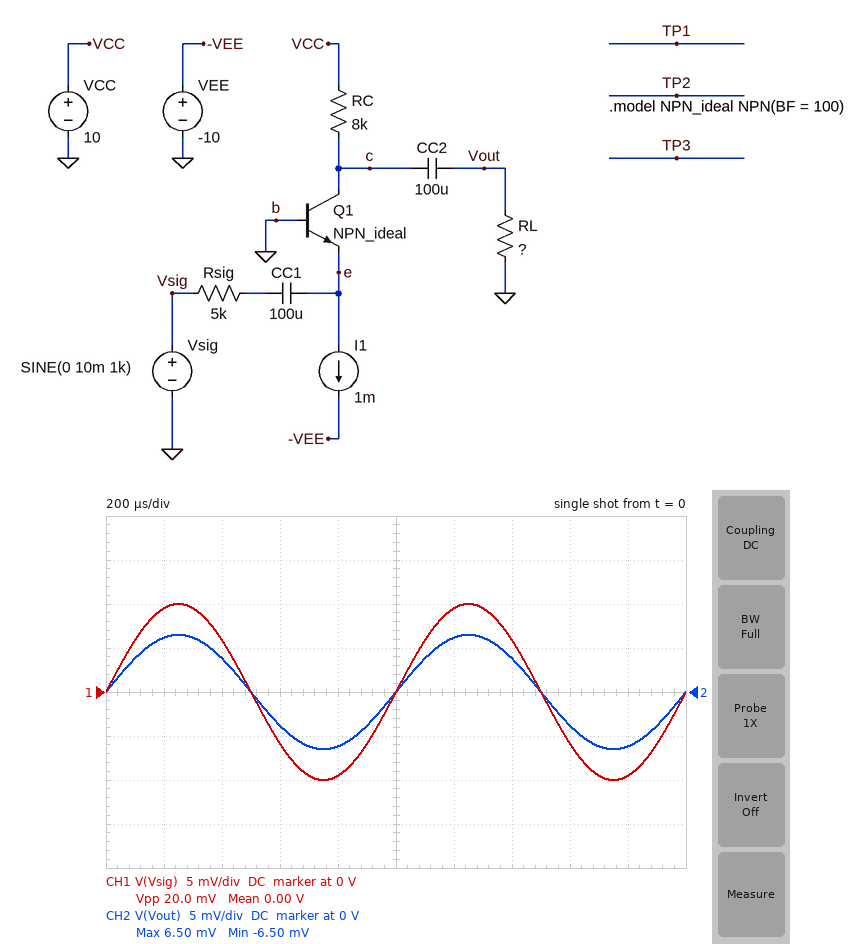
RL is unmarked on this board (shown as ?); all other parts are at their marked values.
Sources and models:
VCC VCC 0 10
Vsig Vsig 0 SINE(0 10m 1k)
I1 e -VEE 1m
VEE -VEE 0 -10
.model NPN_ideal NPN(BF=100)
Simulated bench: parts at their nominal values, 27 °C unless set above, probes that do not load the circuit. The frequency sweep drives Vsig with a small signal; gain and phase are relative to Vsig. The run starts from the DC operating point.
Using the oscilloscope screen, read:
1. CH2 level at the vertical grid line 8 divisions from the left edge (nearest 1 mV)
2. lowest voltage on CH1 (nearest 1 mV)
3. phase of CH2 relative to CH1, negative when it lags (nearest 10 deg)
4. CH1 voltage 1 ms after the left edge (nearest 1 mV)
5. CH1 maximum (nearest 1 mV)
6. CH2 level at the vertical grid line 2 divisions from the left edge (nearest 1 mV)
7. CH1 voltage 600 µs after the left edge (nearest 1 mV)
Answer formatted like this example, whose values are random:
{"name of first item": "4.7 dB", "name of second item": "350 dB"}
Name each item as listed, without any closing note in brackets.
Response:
{"CH2 level at the vertical grid line 8 divisions from the left edge": "-4 mV", "lowest voltage on CH1": "-10 mV", "phase of CH2 relative to CH1, negative when it lags": "0 deg", "CH1 voltage 1 ms after the left edge": "0 V", "CH1 maximum": "10 mV", "CH2 level at the vertical grid line 2 divisions from the left edge": "4 mV", "CH1 voltage 600 µs after the left edge": "-6 mV"}
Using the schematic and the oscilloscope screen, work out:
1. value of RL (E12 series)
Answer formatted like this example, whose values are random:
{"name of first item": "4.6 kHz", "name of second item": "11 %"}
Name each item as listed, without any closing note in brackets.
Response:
{"value of RL": "5.6 kΩ"}
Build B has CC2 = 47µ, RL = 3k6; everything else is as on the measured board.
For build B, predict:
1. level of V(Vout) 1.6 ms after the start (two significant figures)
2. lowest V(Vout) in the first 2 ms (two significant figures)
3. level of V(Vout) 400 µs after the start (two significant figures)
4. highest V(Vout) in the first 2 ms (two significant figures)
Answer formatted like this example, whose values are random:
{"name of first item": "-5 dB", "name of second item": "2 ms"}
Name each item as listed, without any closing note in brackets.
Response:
{"level of V(Vout) 1.6 ms after the start": "-2.9 mV", "lowest V(Vout) in the first 2 ms": "-4.9 mV", "level of V(Vout) 400 µs after the start": "2.9 mV", "highest V(Vout) in the first 2 ms": "4.9 mV"}
